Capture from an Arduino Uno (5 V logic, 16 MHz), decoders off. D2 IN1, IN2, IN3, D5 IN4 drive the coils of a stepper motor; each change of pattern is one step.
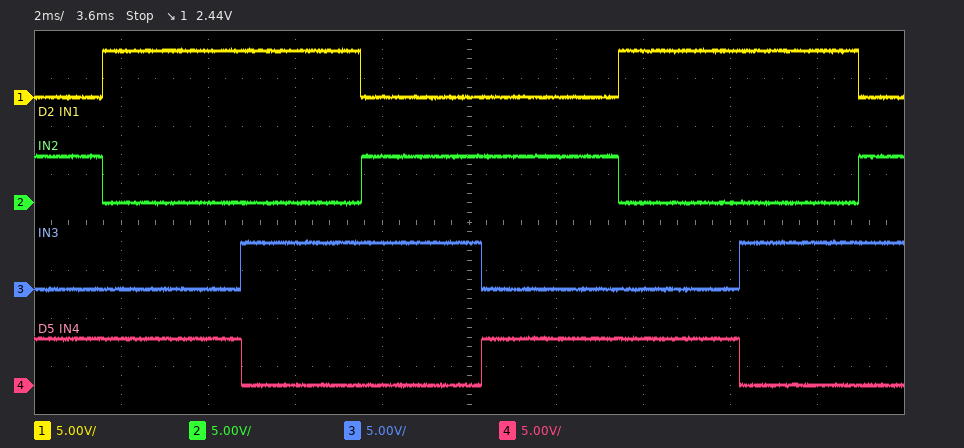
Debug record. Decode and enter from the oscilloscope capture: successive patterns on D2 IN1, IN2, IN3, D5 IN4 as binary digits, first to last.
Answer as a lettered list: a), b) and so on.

a) 0101 1001 1010 0110 0101 1001 1010 0110
